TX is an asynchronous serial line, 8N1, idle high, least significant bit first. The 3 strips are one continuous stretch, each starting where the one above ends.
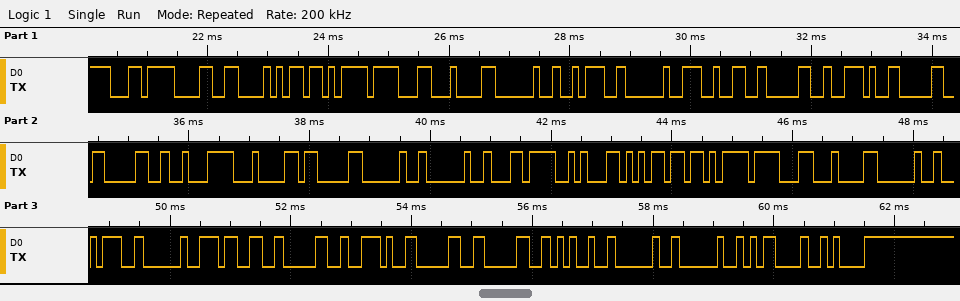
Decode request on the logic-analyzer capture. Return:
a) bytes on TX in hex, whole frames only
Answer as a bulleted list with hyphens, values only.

- 0xEC 0x98 0xA8 0xEB 0x8F 0x84 0x20 0x3A 0x20 0x32 0x30 0x2E 0x30 0x30 0xE2 0x84 0x83 0x20 0x20 0xEC 0x8A 0xB5 0xEB 0x8F 0x84 0x20 0x3A 0x20 0x33 0x30 0x2E 0x30 0x30 0x25 0x20 0x20 0x0D 0x0A
